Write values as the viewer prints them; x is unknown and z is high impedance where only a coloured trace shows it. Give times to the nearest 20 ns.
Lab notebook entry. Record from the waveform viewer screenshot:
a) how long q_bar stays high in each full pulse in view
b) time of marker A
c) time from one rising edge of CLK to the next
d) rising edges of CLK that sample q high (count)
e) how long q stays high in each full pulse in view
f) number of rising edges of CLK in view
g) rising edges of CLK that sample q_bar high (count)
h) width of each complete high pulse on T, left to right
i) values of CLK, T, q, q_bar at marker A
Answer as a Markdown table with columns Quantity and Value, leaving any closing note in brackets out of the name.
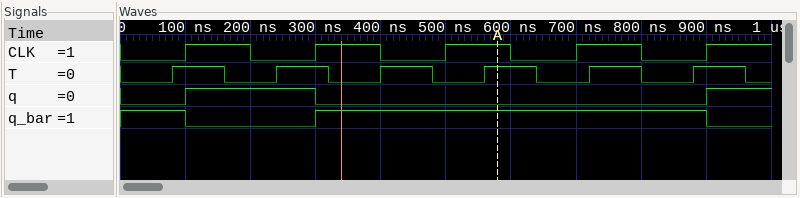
| Quantity | Value |
|---|---|
| how long q_bar stays high in each full pulse in view | 600 ns |
| time of marker A | 580 ns |
| time from one rising edge of CLK to the next | 200 ns |
| rising edges of CLK that sample q high | 1 |
| how long q stays high in each full pulse in view | 200 ns |
| number of rising edges of CLK in view | 5 |
| rising edges of CLK that sample q_bar high | 4 |
| width of each complete high pulse on T, left to right | 80 ns, 80 ns, 80 ns, 80 ns, 80 ns, 80 ns |
| values of CLK, T, q, q_bar at marker A | CLK=1, T=1, q=0, q_bar=1 |
